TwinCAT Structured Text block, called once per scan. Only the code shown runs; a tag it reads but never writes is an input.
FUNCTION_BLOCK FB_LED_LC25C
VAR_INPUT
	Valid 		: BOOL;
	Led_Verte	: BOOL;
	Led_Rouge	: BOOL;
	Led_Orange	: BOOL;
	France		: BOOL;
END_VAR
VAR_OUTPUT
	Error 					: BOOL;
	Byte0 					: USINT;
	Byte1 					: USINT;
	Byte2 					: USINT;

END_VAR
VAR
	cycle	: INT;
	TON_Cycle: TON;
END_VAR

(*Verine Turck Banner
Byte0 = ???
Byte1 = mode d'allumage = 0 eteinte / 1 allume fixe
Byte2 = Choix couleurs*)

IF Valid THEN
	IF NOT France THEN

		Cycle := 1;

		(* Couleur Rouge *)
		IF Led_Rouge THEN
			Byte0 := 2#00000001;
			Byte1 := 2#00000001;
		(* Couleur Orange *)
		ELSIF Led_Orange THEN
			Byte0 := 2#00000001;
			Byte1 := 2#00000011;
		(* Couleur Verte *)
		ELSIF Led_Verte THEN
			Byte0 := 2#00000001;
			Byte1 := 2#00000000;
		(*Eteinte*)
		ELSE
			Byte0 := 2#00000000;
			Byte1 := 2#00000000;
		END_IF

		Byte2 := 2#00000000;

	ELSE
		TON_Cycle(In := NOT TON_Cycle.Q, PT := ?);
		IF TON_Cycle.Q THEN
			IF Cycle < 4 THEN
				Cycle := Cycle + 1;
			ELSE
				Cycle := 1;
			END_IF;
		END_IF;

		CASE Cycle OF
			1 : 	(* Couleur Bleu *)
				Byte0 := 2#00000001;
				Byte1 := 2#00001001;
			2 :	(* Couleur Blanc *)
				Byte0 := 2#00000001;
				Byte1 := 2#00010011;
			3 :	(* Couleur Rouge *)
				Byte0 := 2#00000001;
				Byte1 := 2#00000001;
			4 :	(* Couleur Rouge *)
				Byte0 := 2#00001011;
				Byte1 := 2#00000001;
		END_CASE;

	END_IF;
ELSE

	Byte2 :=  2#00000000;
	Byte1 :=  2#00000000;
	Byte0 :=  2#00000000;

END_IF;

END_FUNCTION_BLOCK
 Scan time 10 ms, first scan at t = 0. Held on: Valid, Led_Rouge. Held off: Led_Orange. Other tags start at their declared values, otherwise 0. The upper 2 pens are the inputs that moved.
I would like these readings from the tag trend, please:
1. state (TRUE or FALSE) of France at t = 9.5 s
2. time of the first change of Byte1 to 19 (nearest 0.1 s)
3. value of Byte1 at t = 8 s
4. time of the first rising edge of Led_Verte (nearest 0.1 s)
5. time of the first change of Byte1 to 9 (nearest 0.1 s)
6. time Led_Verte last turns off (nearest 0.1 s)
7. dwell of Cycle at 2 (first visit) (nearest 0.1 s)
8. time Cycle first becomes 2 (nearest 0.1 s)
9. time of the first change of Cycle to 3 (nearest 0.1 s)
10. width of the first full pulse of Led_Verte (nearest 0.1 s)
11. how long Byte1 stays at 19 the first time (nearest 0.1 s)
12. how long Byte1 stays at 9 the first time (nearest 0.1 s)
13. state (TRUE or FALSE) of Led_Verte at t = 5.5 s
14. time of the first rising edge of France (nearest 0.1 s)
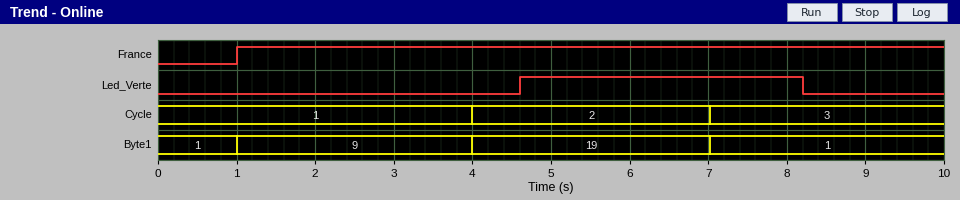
TRUE
4.0 s
1
4.6 s
1.0 s
8.2 s
3.0 s
4.0 s
7.0 s
3.6 s
3.0 s
3.0 s
TRUE
1.0 s
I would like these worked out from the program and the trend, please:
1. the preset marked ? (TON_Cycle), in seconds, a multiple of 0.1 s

3.0 s
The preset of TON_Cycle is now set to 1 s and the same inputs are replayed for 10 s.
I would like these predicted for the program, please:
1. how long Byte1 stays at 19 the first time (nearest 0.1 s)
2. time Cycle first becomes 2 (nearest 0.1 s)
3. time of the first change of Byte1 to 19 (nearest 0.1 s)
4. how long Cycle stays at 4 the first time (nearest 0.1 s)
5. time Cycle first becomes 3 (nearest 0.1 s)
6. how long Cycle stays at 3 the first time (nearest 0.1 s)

1.0 s
2.0 s
2.0 s
1.0 s
3.0 s
1.0 s
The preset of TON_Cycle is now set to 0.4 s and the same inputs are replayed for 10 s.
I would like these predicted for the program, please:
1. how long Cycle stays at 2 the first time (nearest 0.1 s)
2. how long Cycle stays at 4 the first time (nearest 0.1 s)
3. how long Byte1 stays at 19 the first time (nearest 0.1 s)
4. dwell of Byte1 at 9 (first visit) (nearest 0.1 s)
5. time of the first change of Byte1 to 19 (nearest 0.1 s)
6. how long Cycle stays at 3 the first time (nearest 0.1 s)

0.4 s
0.4 s
0.4 s
0.4 s
1.4 s
0.4 s
